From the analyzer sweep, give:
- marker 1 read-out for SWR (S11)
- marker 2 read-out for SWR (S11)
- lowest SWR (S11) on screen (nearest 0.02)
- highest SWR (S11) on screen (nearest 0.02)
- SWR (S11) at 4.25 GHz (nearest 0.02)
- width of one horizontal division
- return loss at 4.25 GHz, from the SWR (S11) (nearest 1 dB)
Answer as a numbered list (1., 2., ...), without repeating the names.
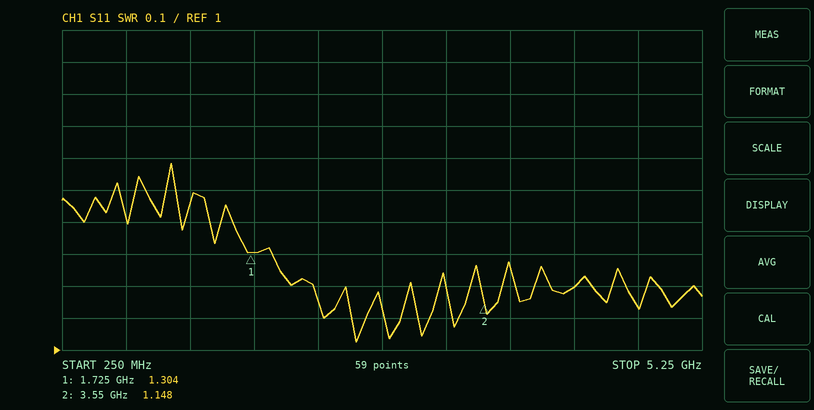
1. 1.304
2. 1.148
3. 1.02
4. 1.58
5. 1.20
6. 500 MHz
7. 21 dB
